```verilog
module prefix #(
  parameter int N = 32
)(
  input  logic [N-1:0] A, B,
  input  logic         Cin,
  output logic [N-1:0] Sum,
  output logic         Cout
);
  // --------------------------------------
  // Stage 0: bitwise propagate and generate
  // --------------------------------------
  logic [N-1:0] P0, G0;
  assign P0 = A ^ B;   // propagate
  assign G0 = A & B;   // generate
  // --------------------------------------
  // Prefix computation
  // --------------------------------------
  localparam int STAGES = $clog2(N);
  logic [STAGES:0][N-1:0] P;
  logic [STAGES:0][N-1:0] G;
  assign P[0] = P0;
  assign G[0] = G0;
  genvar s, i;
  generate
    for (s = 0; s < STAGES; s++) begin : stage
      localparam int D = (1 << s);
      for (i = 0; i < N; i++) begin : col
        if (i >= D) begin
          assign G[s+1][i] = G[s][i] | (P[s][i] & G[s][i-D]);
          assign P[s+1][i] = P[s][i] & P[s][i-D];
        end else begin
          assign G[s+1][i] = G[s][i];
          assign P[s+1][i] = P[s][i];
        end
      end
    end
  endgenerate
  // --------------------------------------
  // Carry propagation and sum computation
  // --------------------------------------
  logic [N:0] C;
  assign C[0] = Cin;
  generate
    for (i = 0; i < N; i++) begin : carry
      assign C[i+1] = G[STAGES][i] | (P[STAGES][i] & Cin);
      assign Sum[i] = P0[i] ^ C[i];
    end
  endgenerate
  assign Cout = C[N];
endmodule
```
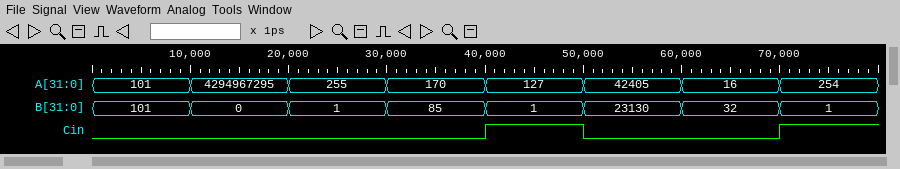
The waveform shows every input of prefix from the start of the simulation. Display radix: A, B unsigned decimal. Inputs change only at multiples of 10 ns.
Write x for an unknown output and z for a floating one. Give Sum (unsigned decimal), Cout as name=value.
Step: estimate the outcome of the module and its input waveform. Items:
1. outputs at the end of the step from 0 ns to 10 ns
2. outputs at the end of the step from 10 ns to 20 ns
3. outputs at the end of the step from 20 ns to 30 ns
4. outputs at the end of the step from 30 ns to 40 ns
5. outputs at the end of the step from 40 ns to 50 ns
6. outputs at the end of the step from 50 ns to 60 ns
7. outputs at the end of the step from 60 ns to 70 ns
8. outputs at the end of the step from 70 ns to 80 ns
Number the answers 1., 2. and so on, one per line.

1. Sum=202, Cout=0
2. Sum=4294967295, Cout=0
3. Sum=256, Cout=0
4. Sum=255, Cout=0
5. Sum=129, Cout=0
6. Sum=65535, Cout=0
7. Sum=48, Cout=0
8. Sum=256, Cout=0
